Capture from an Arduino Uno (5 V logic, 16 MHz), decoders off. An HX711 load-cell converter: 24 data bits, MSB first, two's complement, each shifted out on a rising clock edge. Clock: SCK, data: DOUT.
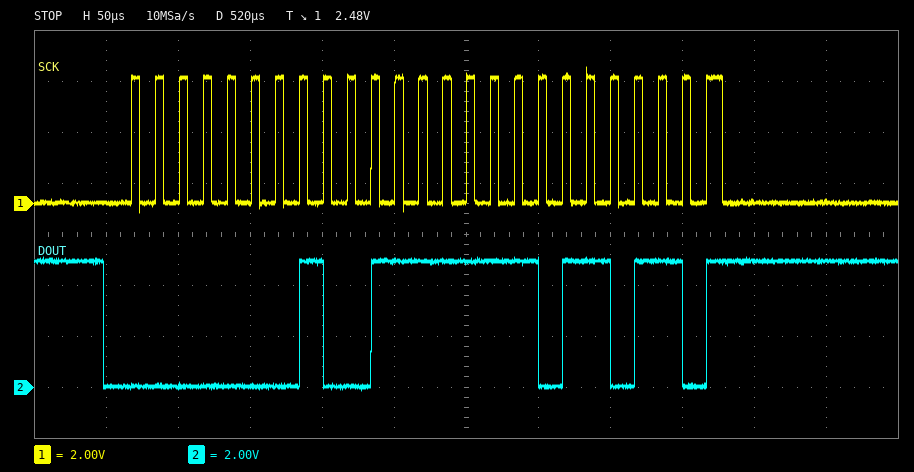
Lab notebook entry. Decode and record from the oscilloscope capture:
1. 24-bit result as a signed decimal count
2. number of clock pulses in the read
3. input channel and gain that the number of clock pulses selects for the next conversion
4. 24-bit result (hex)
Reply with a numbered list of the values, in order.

1. 81846
2. 25
3. channel A, gain 128
4. 0x013FB6
